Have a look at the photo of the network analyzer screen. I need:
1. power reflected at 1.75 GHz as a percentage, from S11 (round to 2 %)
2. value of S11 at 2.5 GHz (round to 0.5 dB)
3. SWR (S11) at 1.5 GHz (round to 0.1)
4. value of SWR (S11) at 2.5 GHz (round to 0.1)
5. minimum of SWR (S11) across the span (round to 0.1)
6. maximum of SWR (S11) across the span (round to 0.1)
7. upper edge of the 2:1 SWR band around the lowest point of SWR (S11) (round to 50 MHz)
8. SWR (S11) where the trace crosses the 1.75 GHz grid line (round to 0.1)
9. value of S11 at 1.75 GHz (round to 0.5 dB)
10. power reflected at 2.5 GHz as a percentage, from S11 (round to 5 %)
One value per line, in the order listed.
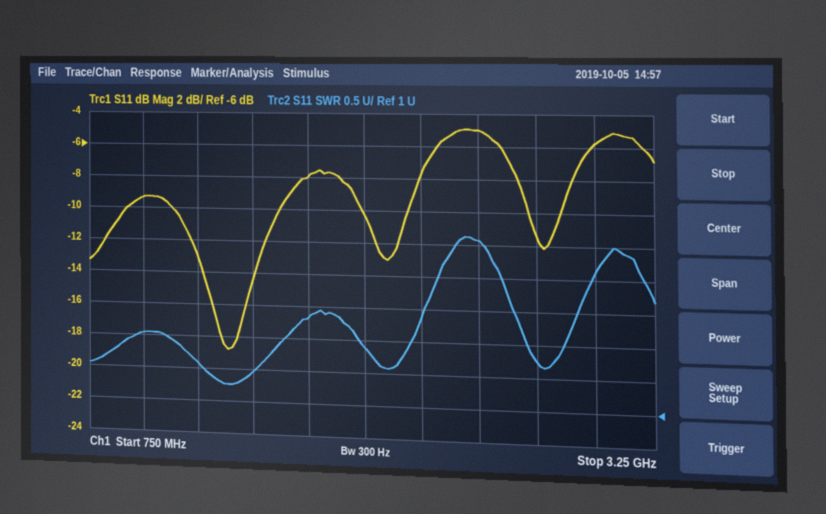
16 %
-5.0 dB
1.5
3.6
1.3
3.6
1.65 GHz
2.3
-8.0 dB
30 %
